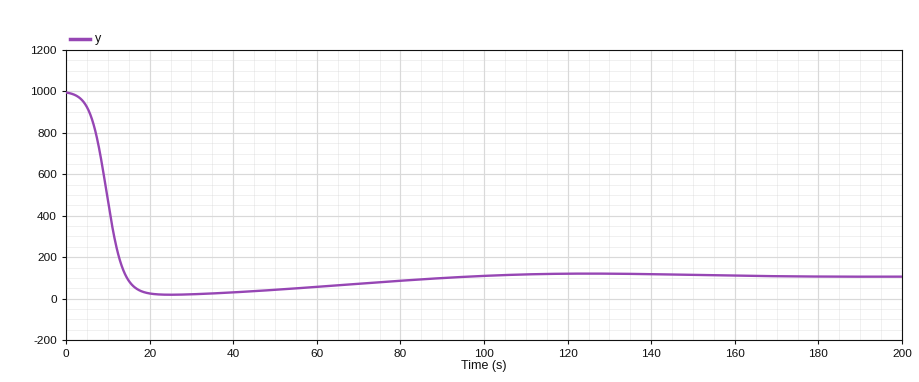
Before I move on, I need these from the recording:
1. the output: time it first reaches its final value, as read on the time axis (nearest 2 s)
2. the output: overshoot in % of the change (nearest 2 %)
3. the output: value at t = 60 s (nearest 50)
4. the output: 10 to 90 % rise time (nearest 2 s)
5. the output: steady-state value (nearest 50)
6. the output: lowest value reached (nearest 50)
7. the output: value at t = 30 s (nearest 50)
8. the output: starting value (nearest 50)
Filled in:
14 s
10 %
50
8 s
100
0
0
1000
